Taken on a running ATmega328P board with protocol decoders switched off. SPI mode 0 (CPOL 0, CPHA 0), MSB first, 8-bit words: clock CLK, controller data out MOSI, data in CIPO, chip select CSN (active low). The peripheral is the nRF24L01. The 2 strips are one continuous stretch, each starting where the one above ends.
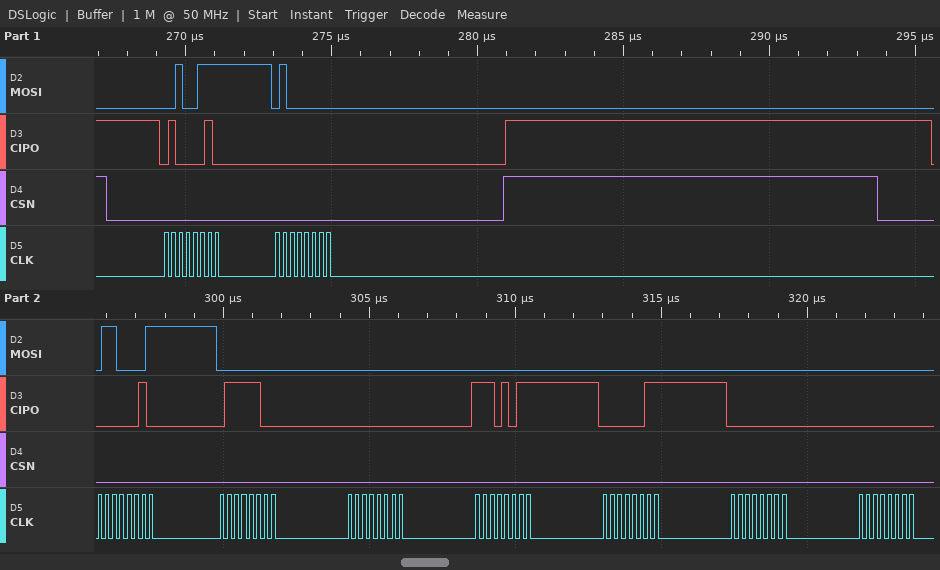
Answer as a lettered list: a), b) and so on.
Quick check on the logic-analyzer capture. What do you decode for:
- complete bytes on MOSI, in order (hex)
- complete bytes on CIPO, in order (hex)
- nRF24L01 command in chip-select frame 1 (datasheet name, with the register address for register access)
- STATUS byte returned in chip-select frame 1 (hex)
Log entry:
a) 27 40 61 00 00 00 00 00 00
b) 42 00 02 7C 00 EB 03 00 00
c) W_REGISTER 0x07
d) 0x42
